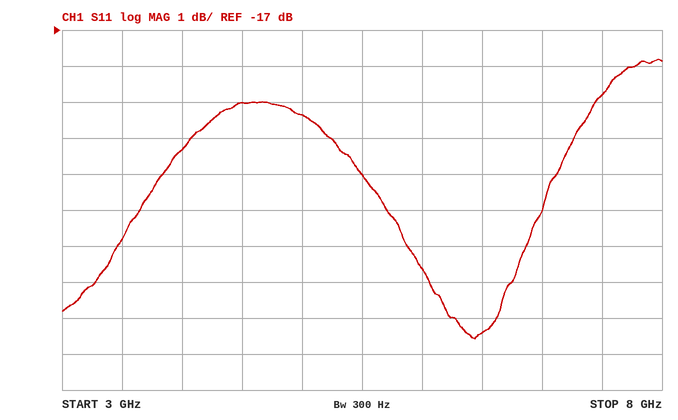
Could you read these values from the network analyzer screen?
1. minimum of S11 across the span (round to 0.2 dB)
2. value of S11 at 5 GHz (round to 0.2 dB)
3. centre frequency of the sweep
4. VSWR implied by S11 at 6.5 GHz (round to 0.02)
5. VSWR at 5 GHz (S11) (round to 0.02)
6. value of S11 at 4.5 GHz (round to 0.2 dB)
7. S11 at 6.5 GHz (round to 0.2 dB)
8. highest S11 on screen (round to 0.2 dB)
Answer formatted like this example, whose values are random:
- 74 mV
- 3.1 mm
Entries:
- -25.6 dB
- -19.4 dB
- 5.5 GHz
- 1.12
- 1.24
- -19.0 dB
- -25.4 dB
- -17.8 dB
